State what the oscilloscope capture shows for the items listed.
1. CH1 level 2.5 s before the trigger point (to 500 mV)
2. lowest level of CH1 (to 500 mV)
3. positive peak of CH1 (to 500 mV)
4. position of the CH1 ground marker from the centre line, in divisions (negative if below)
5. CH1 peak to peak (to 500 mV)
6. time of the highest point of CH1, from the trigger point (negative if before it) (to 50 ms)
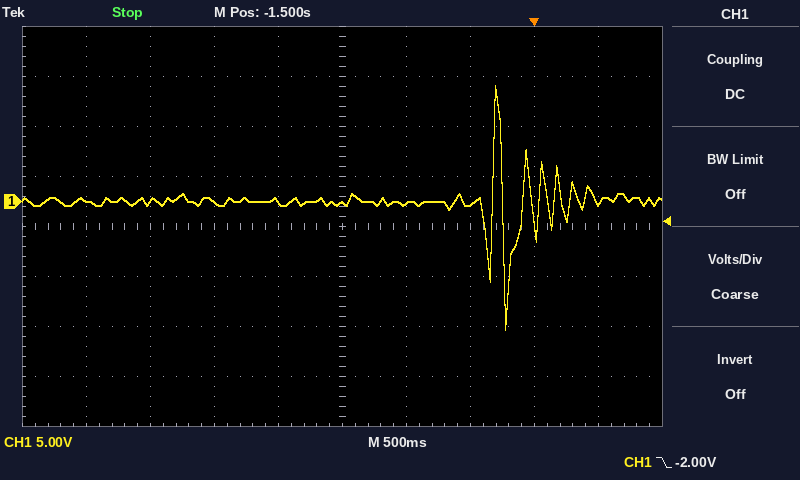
0.0 V
-13.0 V
11.5 V
+0.5 div
24.5 V
-300 ms
